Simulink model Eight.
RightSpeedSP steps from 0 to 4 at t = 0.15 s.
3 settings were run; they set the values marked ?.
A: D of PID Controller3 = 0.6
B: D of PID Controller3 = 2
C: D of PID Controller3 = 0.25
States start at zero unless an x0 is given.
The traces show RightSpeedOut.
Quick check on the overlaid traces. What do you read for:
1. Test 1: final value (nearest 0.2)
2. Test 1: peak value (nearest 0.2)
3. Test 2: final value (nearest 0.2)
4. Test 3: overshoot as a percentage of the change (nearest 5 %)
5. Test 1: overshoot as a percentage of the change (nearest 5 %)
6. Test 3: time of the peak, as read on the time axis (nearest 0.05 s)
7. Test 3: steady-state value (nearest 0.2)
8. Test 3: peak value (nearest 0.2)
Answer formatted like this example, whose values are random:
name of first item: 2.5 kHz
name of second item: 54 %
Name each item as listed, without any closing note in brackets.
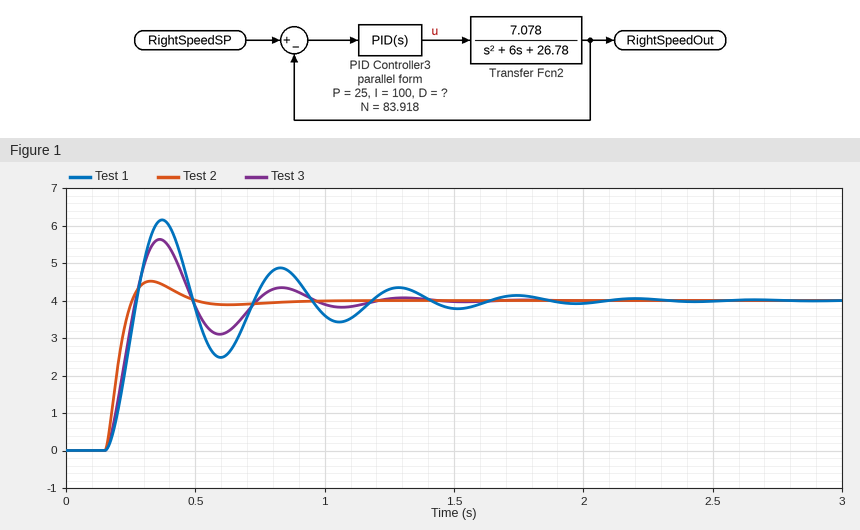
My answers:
Test 1: final value: 4.0
Test 1: peak value: 6.2
Test 2: final value: 4.0
Test 3: overshoot as a percentage of the change: 40 %
Test 1: overshoot as a percentage of the change: 55 %
Test 3: time of the peak, as read on the time axis: 0.35 s
Test 3: steady-state value: 4.0
Test 3: peak value: 5.6
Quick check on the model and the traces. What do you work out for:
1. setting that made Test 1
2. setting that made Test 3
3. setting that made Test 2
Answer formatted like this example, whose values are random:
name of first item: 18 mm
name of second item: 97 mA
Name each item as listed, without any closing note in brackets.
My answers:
setting that made Test 1: C
setting that made Test 3: A
setting that made Test 2: B
